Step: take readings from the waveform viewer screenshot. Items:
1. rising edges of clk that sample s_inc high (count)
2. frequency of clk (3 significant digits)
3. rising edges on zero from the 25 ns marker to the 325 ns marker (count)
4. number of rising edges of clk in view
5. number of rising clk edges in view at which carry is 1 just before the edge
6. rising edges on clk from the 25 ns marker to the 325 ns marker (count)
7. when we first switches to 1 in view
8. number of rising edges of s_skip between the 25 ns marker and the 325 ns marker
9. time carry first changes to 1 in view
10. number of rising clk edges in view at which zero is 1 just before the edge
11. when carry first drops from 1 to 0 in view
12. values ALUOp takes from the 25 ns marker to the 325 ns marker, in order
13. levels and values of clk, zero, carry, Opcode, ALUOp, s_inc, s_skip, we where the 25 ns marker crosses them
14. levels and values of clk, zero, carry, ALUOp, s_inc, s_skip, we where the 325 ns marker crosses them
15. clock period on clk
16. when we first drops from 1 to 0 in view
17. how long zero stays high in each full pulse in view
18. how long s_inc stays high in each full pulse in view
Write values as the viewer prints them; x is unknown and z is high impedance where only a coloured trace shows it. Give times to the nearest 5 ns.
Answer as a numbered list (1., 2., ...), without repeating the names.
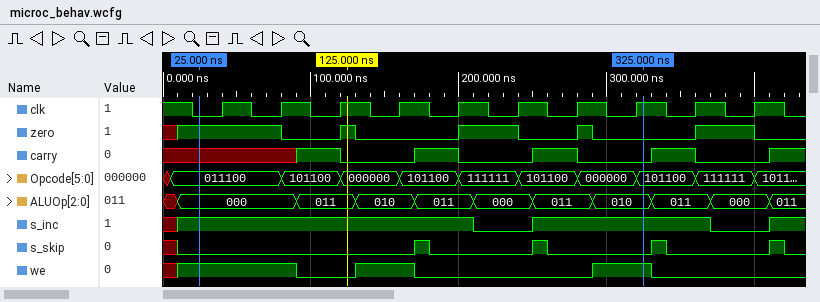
1. 8
2. 25.0 MHz
3. 3
4. 10
5. 4
6. 8
7. 10 ns
8. 2
9. 90 ns
10. 4
11. 120 ns
12. 000, 011, 010, 011, 000, 011, 010
13. clk=0, zero=1, carry=x, Opcode=011100, ALUOp=000, s_inc=1, s_skip=0, we=1
14. clk=1, zero=0, carry=0, ALUOp=010, s_inc=1, s_skip=0, we=1
15. 40 ns
16. 90 ns
17. 10 ns, 40 ns, 10 ns, 40 ns
18. 120 ns
